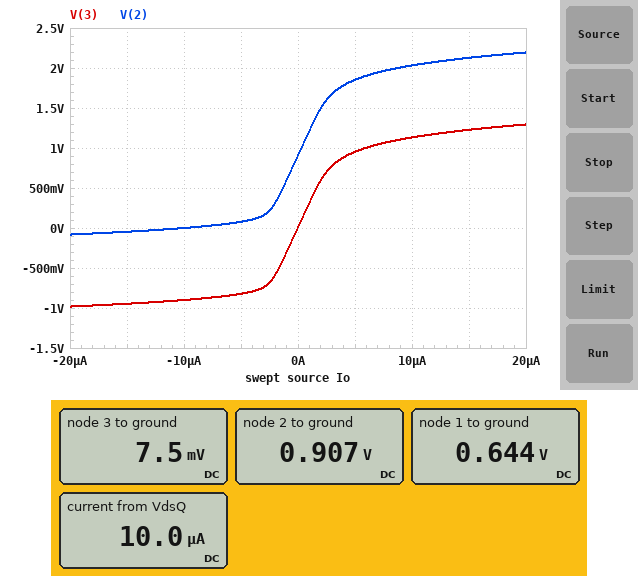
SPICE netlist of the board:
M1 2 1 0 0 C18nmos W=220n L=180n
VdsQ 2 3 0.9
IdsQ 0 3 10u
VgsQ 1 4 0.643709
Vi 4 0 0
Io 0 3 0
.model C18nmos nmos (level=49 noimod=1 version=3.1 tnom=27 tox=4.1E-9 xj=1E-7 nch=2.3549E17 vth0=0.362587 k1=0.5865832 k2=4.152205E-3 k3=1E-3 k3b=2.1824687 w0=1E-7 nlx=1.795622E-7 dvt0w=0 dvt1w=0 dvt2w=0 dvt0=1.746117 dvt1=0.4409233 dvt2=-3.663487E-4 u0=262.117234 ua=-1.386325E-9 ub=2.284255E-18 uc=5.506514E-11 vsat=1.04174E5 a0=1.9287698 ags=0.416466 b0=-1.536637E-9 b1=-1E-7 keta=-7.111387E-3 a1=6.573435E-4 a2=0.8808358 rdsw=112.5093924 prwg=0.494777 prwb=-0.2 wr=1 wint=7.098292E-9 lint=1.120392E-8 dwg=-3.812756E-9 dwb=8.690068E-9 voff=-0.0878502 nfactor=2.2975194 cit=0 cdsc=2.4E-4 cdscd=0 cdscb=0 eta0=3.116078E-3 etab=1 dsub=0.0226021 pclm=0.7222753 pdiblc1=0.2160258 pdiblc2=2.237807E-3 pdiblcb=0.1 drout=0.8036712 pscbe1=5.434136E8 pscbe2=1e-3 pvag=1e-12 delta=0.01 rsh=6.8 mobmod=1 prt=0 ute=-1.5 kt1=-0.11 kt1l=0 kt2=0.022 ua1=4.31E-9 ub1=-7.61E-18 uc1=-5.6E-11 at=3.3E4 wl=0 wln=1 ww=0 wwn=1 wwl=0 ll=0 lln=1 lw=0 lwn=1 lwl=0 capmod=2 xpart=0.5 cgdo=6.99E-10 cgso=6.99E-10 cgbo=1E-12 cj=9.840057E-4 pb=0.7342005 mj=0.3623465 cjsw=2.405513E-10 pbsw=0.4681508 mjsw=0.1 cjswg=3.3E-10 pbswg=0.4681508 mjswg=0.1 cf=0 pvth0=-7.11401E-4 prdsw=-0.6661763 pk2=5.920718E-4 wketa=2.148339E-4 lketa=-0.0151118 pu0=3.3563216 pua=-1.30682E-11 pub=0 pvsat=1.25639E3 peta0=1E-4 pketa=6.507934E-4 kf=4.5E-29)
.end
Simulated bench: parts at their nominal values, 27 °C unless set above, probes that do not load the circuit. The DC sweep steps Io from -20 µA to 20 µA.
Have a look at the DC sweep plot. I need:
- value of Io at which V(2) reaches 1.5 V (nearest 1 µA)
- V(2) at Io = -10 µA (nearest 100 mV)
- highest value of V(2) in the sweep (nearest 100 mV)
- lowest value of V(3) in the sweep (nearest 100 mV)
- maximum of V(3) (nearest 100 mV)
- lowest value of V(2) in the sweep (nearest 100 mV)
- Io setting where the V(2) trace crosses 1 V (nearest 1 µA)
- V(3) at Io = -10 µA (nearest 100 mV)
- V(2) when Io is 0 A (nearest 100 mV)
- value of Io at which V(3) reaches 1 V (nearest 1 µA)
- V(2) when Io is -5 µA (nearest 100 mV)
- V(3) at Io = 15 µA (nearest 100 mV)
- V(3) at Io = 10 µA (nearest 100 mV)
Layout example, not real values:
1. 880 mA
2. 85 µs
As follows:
1. 2 µA
2. 0 V
3. 2.2 V
4. -1.0 V
5. 1.3 V
6. -100 mV
7. 0 A
8. -900 mV
9. 900 mV
10. 6 µA
11. 100 mV
12. 1.2 V
13. 1.1 V
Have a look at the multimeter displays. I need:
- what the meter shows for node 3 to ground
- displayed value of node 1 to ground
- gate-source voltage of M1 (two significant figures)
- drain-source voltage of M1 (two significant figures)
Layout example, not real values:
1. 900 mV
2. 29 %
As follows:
1. 7.5 mV
2. 0.644 V
3. 640 mV
4. 910 mV
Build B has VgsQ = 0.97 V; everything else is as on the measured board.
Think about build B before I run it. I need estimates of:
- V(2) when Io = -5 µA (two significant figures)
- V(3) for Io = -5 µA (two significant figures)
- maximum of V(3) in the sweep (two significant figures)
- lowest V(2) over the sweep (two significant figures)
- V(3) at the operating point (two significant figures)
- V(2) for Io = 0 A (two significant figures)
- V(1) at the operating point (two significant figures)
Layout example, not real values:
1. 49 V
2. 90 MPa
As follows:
1. 20 mV
2. -880 mV
3. -740 mV
4. -38 mV
5. -860 mV
6. 42 mV
7. 970 mV
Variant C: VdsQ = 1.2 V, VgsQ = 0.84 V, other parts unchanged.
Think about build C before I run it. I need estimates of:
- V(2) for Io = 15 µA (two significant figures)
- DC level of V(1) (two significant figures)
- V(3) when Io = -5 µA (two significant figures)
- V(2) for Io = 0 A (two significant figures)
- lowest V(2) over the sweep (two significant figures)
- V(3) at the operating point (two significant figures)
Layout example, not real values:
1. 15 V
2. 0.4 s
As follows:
1. 230 mV
2. 840 mV
3. -1.2 V
4. 58 mV
5. -48 mV
6. -1.1 V
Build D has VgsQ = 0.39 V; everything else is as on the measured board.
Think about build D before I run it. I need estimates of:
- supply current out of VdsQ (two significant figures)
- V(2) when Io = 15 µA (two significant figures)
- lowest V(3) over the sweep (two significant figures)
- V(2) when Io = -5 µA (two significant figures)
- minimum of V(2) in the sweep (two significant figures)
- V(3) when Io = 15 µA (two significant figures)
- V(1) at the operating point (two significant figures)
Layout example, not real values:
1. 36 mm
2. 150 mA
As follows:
1. 10 µA
2. 3.2 V
3. -1.1 V
4. 2.6 V
5. -180 mV
6. 2.3 V
7. 390 mV
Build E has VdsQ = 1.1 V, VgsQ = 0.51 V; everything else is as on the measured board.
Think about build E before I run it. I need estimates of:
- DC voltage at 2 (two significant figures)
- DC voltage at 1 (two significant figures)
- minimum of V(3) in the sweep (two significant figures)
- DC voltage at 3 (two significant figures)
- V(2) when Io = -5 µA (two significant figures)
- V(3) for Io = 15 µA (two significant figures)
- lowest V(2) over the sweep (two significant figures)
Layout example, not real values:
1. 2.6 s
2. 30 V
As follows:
1. 2.2 V
2. 510 mV
3. -1.2 V
4. 1.1 V
5. 2.0 V
6. 1.4 V
7. -130 mV
